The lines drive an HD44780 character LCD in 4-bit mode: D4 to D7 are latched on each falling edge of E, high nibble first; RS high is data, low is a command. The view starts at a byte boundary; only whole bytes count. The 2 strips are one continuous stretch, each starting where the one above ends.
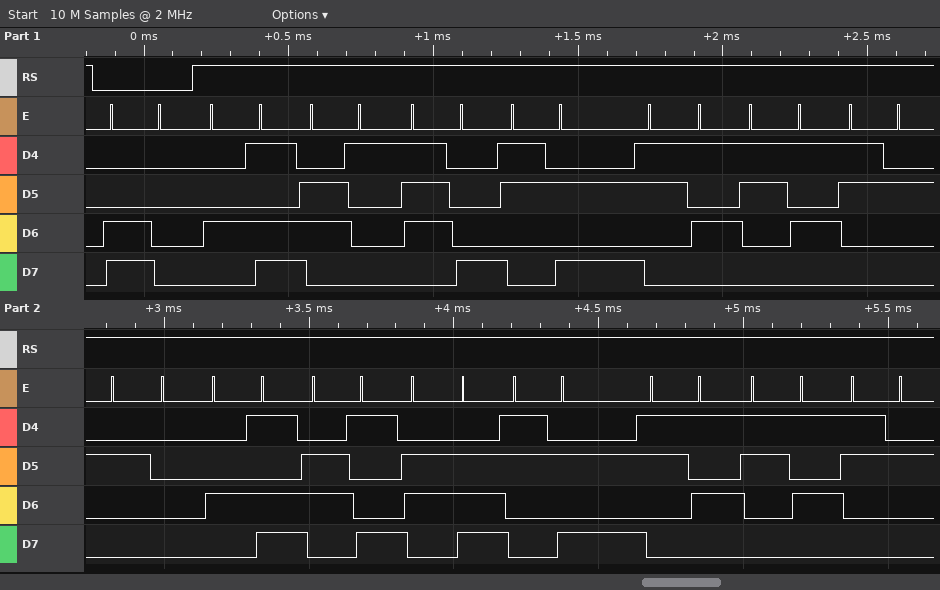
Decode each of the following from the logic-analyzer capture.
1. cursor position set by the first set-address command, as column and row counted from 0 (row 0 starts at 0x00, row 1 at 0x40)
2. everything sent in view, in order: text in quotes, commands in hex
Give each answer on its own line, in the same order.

column 0, row 1
0xC0 "Max:552 Min:552"
